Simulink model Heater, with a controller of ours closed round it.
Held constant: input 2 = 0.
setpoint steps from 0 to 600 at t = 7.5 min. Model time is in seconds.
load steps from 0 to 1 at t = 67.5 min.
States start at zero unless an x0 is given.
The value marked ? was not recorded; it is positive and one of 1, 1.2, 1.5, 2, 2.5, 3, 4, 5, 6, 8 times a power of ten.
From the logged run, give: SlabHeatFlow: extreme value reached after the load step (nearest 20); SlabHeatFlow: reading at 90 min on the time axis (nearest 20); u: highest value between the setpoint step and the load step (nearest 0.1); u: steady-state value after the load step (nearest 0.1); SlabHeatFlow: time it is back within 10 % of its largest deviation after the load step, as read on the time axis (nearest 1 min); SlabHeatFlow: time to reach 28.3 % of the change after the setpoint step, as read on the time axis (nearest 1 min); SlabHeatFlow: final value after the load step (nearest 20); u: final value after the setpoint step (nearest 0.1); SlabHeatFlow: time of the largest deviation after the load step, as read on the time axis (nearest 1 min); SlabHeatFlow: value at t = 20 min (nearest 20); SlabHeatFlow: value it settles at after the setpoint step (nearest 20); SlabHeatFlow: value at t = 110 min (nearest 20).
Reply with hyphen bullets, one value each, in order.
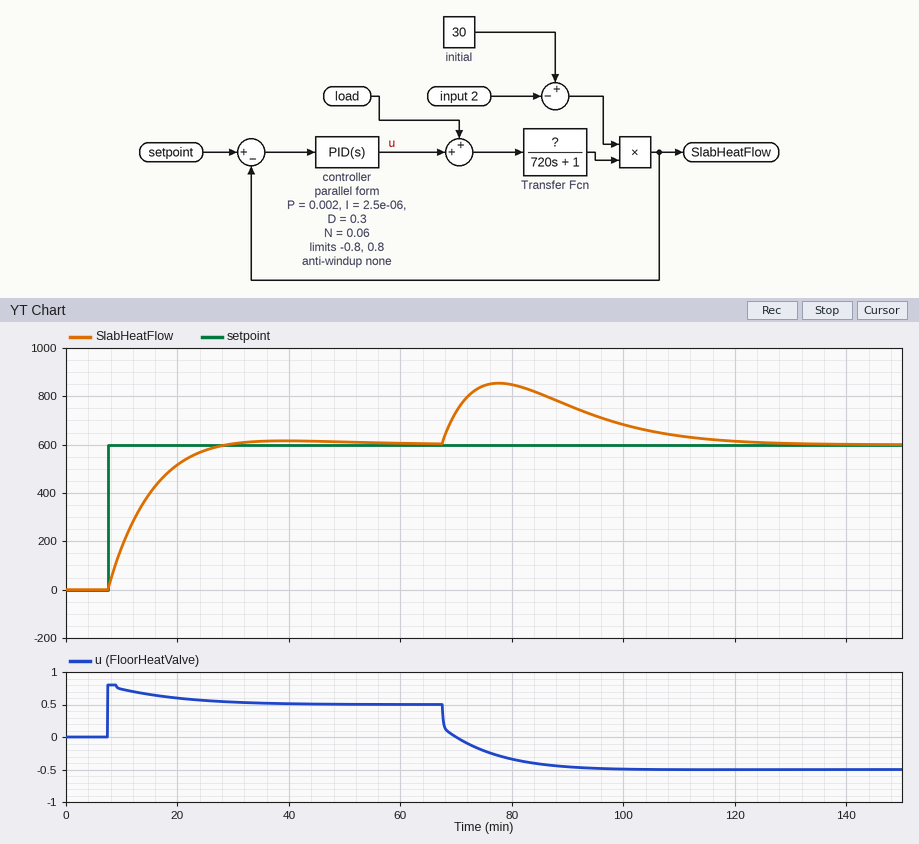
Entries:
- 860
- 760
- 0.8
- -0.5
- 114 min
- 10 min
- 600
- 0.5
- 78 min
- 520
- 600
- 640
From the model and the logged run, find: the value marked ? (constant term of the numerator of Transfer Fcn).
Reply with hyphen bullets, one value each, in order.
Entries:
- 40
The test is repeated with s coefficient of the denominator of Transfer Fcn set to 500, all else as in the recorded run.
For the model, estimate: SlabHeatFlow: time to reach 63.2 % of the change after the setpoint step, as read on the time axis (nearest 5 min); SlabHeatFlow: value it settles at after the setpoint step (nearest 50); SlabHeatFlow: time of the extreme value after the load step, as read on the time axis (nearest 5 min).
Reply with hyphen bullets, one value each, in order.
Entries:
- 15 min
- 600
- 75 min
